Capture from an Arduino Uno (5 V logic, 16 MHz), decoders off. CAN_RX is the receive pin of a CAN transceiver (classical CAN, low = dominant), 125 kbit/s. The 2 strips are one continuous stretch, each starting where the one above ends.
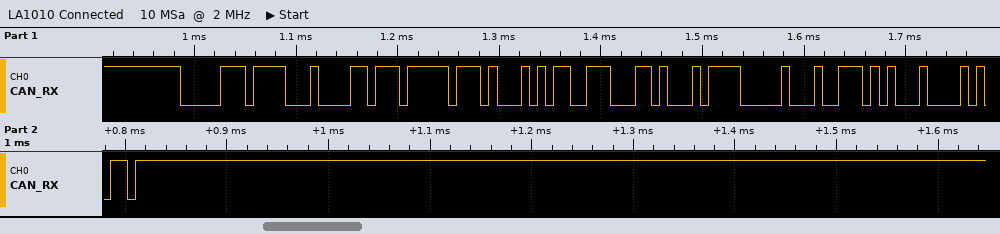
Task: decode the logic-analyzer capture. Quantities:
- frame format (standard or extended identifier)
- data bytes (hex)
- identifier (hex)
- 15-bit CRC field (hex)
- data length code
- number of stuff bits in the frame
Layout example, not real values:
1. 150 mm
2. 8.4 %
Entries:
1. standard
2. 6E FF 45 67 1A 2F 00 9D
3. 0x06F
4. 0x2215
5. 8
6. 3
